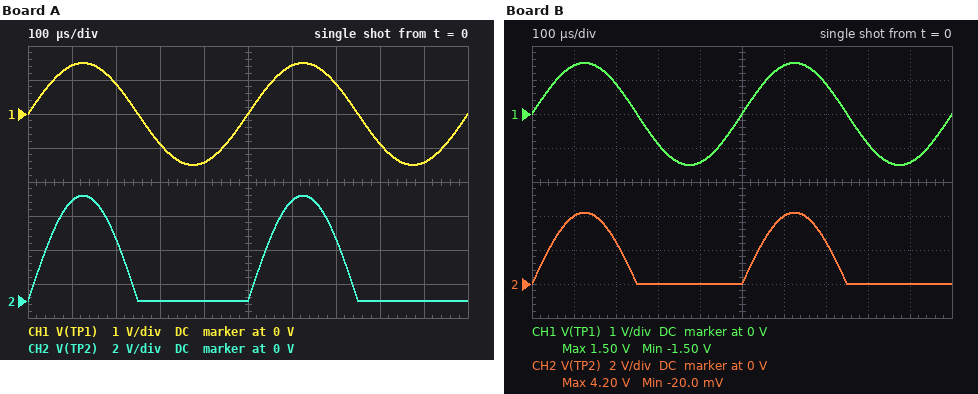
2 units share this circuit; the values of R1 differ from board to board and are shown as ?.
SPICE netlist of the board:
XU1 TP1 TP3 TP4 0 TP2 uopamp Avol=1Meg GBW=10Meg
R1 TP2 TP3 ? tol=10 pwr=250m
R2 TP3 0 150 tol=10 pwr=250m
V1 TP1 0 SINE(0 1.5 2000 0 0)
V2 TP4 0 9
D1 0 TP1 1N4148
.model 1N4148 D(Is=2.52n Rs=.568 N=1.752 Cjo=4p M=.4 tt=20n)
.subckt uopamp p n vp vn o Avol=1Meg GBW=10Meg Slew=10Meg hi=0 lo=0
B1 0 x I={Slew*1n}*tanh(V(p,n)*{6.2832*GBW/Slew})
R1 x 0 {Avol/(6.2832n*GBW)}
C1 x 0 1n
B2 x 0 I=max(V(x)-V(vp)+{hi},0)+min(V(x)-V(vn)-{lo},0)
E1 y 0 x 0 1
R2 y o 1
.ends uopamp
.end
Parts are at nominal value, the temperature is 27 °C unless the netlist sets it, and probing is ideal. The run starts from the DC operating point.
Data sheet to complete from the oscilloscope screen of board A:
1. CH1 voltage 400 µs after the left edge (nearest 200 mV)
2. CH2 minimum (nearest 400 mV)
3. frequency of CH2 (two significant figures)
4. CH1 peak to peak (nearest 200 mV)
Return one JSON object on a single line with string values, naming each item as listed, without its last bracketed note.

{"CH1 voltage 400 µs after the left edge": "-1.4 V", "CH2 minimum": "0 V", "frequency of CH2": "2.0 kHz", "CH1 peak to peak": "3.0 V"}
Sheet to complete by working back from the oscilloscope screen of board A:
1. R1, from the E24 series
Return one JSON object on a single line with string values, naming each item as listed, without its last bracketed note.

{"R1, from the E24 series": "470 Ω"}
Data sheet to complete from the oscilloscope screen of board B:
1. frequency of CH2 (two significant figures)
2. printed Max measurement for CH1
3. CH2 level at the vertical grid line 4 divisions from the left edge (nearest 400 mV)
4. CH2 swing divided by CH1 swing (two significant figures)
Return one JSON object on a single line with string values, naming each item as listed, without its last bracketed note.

{"frequency of CH2": "2.0 kHz", "printed Max measurement for CH1": "1.50 V", "CH2 level at the vertical grid line 4 divisions from the left edge": "0 V", "CH2 swing divided by CH1 swing": "1.4"}
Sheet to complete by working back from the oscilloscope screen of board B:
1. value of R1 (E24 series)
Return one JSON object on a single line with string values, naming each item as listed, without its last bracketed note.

{"value of R1": "270 Ω"}
